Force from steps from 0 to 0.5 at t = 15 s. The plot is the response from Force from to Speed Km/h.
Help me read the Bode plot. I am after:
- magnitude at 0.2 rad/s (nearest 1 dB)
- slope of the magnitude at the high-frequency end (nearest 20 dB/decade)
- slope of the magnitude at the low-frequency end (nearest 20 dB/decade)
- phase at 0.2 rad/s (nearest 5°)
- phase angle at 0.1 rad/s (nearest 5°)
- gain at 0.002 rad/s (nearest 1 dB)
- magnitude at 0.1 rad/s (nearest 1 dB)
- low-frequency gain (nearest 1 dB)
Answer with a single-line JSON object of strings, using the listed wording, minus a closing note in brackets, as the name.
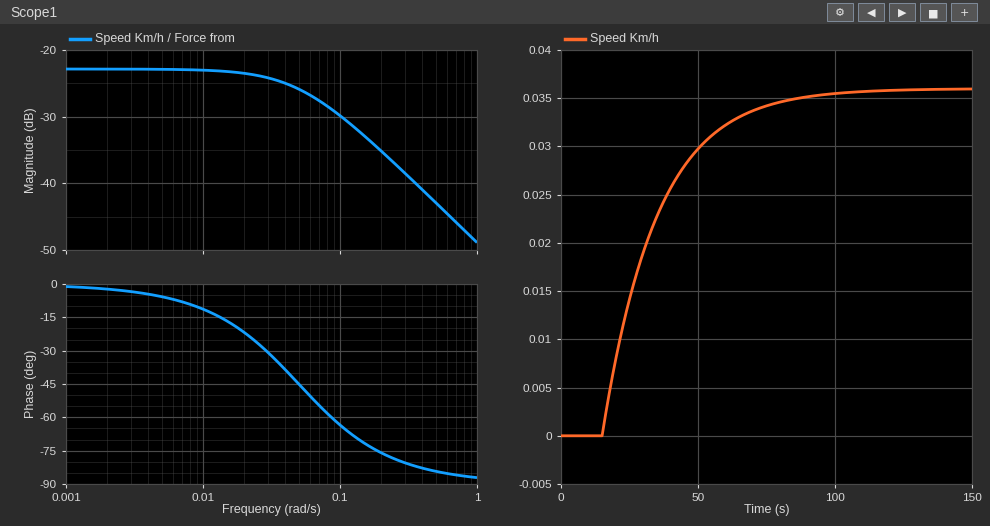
{"magnitude at 0.2 rad/s": "-35 dB", "slope of the magnitude at the high-frequency end": "-20 dB/decade", "slope of the magnitude at the low-frequency end": "0 dB/decade", "phase at 0.2 rad/s": "-75°", "phase angle at 0.1 rad/s": "-65°", "gain at 0.002 rad/s": "-23 dB", "magnitude at 0.1 rad/s": "-30 dB", "low-frequency gain": "-23 dB"}
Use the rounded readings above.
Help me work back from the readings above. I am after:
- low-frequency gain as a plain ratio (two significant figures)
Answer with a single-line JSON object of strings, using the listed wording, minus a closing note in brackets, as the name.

{"low-frequency gain as a plain ratio": "0.071"}
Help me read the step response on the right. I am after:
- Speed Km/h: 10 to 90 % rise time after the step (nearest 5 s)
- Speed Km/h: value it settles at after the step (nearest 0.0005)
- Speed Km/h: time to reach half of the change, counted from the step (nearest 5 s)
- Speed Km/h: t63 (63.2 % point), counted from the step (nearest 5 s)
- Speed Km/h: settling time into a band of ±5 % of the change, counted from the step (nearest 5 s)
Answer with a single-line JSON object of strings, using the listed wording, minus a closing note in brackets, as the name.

{"Speed Km/h: 10 to 90 % rise time after the step": "45 s", "Speed Km/h: value it settles at after the step": "0.0360", "Speed Km/h: time to reach half of the change, counted from the step": "15 s", "Speed Km/h: t63 (63.2 % point), counted from the step": "20 s", "Speed Km/h: settling time into a band of ±5 % of the change, counted from the step": "60 s"}
